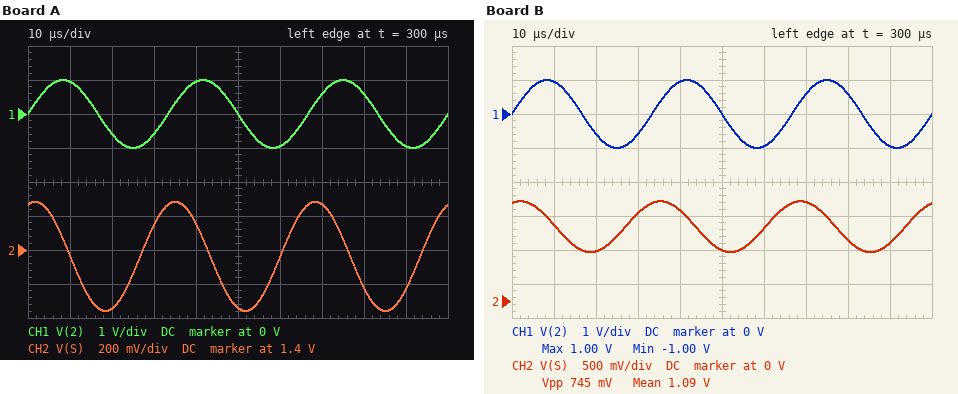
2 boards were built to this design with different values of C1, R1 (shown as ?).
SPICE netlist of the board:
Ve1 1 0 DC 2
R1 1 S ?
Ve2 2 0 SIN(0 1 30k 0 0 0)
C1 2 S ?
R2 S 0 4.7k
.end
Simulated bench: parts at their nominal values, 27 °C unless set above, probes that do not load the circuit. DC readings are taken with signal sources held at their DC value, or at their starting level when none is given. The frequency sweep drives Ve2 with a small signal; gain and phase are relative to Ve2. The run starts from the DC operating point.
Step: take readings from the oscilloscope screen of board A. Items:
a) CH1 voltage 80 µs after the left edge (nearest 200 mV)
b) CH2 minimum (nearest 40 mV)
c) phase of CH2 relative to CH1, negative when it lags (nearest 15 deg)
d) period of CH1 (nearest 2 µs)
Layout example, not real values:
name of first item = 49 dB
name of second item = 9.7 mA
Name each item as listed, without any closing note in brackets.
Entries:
CH1 voltage 80 µs after the left edge = 600 mV
CH2 minimum = 1.04 V
phase of CH2 relative to CH1, negative when it lags = 75 deg
period of CH1 = 34 µs
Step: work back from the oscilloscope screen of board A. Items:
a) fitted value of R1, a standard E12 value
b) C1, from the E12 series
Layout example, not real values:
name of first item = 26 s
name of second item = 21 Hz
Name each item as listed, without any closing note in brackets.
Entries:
fitted value of R1, a standard E12 value = 2.2 kΩ
C1, from the E12 series = 1.2 nF
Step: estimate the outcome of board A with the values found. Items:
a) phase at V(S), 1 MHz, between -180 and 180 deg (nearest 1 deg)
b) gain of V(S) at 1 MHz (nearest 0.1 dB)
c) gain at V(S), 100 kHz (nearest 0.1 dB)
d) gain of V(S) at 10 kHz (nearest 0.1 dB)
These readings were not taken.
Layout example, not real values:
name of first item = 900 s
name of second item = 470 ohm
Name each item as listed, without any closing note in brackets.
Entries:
phase at V(S), 1 MHz, between -180 and 180 deg = 5 deg
gain of V(S) at 1 MHz = 0 dB
gain at V(S), 100 kHz = -2.5 dB
gain of V(S) at 10 kHz = -19.0 dB
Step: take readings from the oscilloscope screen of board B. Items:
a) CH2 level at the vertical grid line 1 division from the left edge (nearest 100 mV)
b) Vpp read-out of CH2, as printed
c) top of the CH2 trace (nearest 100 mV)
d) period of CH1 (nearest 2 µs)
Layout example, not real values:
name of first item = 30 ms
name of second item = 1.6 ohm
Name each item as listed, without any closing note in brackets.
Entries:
CH2 level at the vertical grid line 1 division from the left edge = 1.1 V
Vpp read-out of CH2, as printed = 745 mV
top of the CH2 trace = 1.5 V
period of CH1 = 34 µs
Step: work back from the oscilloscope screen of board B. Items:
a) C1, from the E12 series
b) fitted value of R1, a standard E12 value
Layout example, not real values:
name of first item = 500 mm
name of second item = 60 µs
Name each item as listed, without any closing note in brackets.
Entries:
C1, from the E12 series = 1 nF
fitted value of R1, a standard E12 value = 3.9 kΩ
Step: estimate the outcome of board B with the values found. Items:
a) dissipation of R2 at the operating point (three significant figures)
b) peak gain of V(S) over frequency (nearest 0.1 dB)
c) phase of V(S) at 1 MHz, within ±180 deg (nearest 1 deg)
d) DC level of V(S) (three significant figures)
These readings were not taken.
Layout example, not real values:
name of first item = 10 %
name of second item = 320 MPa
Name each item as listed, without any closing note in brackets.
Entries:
dissipation of R2 at the operating point = 254 µW
peak gain of V(S) over frequency = 0 dB
phase of V(S) at 1 MHz, within ±180 deg = 4 deg
DC level of V(S) = 1.09 V
